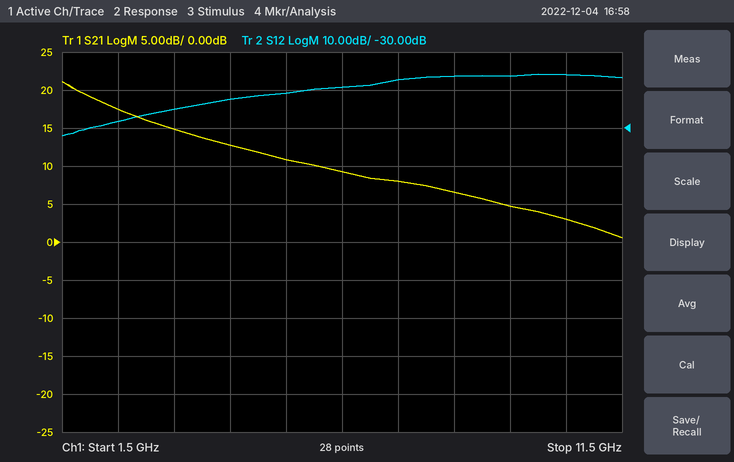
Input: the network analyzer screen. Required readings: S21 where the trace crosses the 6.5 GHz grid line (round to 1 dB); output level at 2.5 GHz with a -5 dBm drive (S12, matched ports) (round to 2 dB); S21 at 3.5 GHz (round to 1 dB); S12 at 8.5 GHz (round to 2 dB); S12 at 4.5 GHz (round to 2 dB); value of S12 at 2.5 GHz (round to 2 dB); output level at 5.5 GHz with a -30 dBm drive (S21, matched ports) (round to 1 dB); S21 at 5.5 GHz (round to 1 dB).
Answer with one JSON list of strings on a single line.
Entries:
["9 dB", "-34 dBm", "15 dB", "-16 dB", "-22 dB", "-28 dB", "-19 dBm", "11 dB"]
